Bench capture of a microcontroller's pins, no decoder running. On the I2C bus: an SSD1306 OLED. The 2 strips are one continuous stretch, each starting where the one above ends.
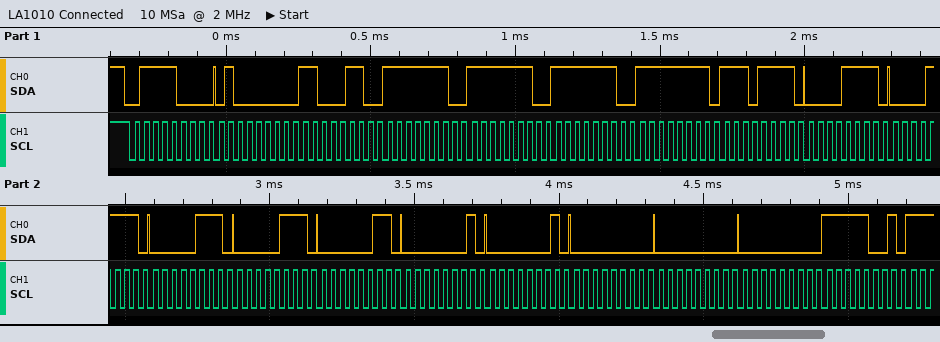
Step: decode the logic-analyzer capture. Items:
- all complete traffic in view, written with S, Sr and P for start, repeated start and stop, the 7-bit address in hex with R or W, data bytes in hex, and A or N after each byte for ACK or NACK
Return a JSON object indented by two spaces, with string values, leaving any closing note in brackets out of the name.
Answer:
{
  "all complete traffic in view, written with S, Sr and P for start, repeated start and stop, the 7-bit address in hex with R or W, data bytes in hex, and A or N after each byte for ACK or NACK": "S 3CW A 40 A C6 A FE A FE A FE A FF A EF A 0F A 0F A 07 A 07 A 03 A 01 A 01 A 00 A 00 A 00 A F9 A"
}
